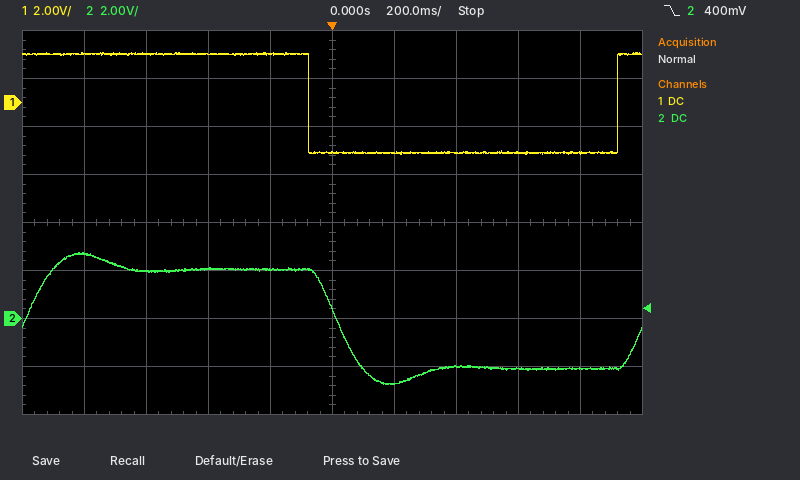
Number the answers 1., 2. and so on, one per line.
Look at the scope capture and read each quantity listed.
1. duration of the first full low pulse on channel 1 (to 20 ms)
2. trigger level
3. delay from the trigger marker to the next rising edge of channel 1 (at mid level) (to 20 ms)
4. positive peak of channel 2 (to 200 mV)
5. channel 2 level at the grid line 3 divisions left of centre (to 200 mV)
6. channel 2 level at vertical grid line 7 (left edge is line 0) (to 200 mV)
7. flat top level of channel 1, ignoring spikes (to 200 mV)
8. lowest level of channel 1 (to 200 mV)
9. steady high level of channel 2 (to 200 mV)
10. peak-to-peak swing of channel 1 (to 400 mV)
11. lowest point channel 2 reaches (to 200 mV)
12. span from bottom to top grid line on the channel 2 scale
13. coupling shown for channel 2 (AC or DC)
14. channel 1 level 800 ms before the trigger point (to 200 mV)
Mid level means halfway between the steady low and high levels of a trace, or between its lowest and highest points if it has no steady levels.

1. 1.00 s
2. 400 mV
3. 920 ms
4. 2.8 V
5. 2.0 V
6. -2.0 V
7. 2.0 V
8. -2.2 V
9. 2.0 V
10. 4.4 V
11. -2.8 V
12. 16 V
13. DC
14. 2.0 V
